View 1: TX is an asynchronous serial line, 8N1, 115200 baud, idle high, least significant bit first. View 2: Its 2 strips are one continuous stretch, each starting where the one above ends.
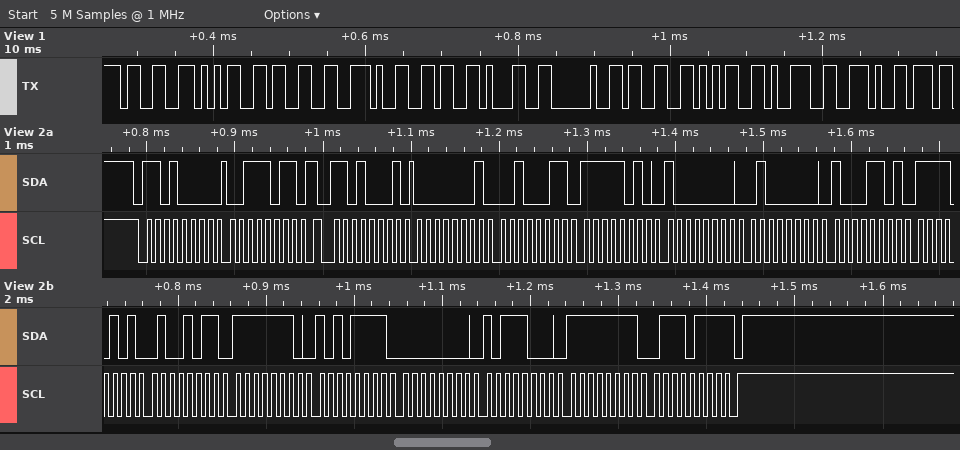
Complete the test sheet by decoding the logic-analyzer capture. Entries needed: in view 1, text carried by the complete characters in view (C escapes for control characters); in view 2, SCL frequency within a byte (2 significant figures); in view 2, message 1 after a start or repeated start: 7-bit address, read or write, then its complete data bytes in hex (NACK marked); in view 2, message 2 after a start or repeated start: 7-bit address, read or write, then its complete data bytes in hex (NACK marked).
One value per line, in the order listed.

"353.61 359."
100 kHz
0x68 write: 3B
0x68 read: 01 23 FA 80 40 8D F5 4B FE AF 00 B8 FF 77 NACK
